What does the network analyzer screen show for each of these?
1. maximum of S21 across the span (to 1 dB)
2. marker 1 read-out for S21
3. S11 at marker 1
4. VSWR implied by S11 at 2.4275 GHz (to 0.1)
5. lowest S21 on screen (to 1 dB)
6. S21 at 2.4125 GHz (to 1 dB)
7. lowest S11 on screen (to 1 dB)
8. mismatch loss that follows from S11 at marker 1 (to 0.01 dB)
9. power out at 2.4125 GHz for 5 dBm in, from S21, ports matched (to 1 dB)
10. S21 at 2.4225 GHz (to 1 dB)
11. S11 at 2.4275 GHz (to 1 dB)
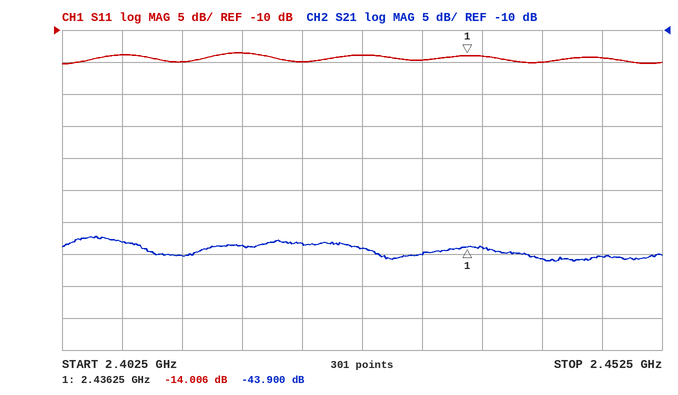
-42 dB
-43.900 dB
-14.006 dB
1.5
-46 dB
-45 dB
-15 dB
0.18 dB
-40 dBm
-43 dB
-14 dB
